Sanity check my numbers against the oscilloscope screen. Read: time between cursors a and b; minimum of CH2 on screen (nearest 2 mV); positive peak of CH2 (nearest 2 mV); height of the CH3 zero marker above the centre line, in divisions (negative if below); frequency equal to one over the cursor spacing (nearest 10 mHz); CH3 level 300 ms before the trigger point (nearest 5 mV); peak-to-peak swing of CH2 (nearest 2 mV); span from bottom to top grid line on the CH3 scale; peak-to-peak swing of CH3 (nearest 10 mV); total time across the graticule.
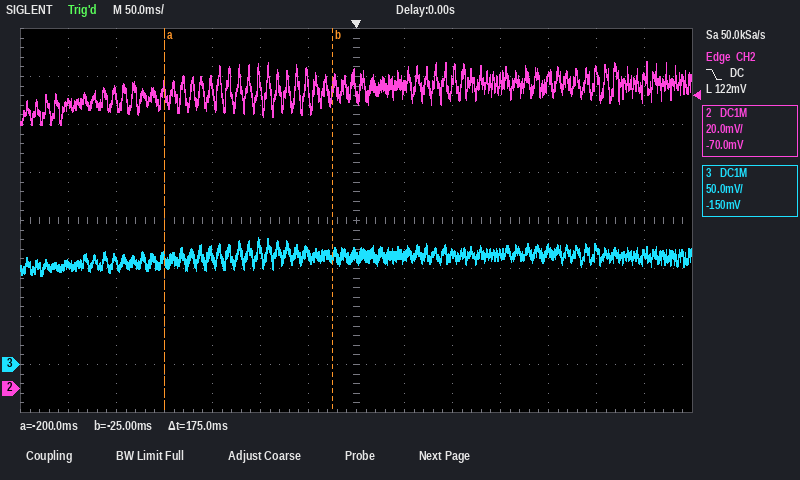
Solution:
175 ms
110 mV
136 mV
-3.0 div
5.71 Hz
105 mV
26 mV
400 mV
40 mV
700 ms
